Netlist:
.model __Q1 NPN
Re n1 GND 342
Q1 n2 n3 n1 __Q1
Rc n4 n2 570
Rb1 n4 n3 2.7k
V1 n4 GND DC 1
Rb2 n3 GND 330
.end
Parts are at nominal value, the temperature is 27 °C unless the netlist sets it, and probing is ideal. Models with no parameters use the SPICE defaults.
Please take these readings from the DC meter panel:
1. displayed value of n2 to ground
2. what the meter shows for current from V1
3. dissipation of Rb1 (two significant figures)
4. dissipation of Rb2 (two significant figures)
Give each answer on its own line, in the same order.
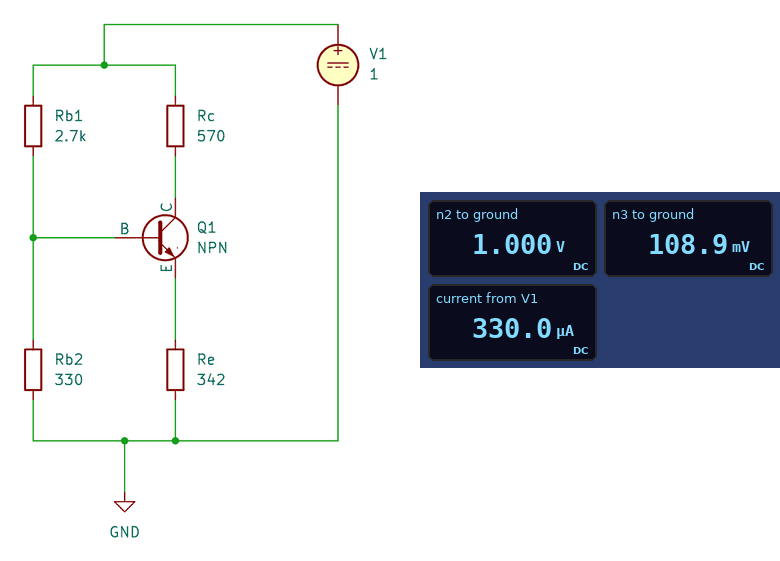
1.000 V
330.0 µA
290 µW
36 µW
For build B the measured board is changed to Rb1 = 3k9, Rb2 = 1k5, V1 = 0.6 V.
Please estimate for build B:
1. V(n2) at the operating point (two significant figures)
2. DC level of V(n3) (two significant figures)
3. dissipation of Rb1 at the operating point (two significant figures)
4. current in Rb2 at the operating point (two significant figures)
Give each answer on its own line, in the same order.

600 mV
170 mV
48 µW
110 µA
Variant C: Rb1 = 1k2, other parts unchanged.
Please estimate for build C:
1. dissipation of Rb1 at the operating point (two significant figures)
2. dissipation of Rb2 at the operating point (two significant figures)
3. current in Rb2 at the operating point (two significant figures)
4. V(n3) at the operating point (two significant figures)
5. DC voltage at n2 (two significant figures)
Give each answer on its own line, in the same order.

510 µW
140 µW
650 µA
220 mV
1.0 V
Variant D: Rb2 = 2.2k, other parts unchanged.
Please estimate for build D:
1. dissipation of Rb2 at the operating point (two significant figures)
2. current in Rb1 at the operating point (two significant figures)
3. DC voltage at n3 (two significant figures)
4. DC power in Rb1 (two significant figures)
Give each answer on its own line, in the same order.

92 µW
200 µA
450 mV
110 µW
